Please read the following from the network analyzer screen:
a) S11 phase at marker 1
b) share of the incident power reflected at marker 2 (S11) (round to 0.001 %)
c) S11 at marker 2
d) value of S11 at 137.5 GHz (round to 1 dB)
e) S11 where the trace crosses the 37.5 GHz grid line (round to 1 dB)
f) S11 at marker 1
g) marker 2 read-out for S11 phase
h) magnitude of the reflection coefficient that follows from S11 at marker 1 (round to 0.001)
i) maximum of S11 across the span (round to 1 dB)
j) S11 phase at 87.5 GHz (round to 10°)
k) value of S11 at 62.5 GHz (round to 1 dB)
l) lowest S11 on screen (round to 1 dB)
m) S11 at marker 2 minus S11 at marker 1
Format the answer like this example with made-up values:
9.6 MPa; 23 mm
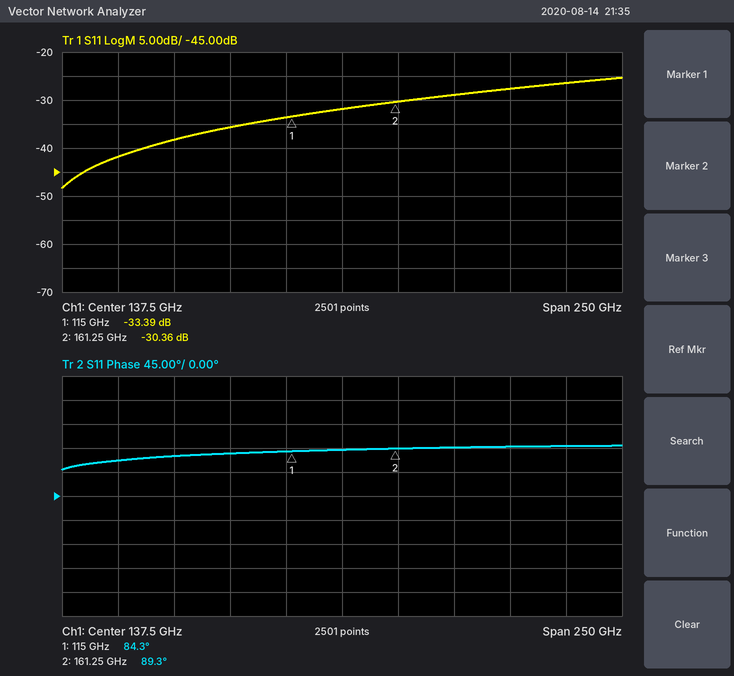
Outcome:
84.3°; 0.092 %; -30.36 dB; -32 dB; -42 dB; -33.39 dB; 89.3°; 0.021; -25 dB; 80°; -38 dB; -48 dB; 3.03 dB
